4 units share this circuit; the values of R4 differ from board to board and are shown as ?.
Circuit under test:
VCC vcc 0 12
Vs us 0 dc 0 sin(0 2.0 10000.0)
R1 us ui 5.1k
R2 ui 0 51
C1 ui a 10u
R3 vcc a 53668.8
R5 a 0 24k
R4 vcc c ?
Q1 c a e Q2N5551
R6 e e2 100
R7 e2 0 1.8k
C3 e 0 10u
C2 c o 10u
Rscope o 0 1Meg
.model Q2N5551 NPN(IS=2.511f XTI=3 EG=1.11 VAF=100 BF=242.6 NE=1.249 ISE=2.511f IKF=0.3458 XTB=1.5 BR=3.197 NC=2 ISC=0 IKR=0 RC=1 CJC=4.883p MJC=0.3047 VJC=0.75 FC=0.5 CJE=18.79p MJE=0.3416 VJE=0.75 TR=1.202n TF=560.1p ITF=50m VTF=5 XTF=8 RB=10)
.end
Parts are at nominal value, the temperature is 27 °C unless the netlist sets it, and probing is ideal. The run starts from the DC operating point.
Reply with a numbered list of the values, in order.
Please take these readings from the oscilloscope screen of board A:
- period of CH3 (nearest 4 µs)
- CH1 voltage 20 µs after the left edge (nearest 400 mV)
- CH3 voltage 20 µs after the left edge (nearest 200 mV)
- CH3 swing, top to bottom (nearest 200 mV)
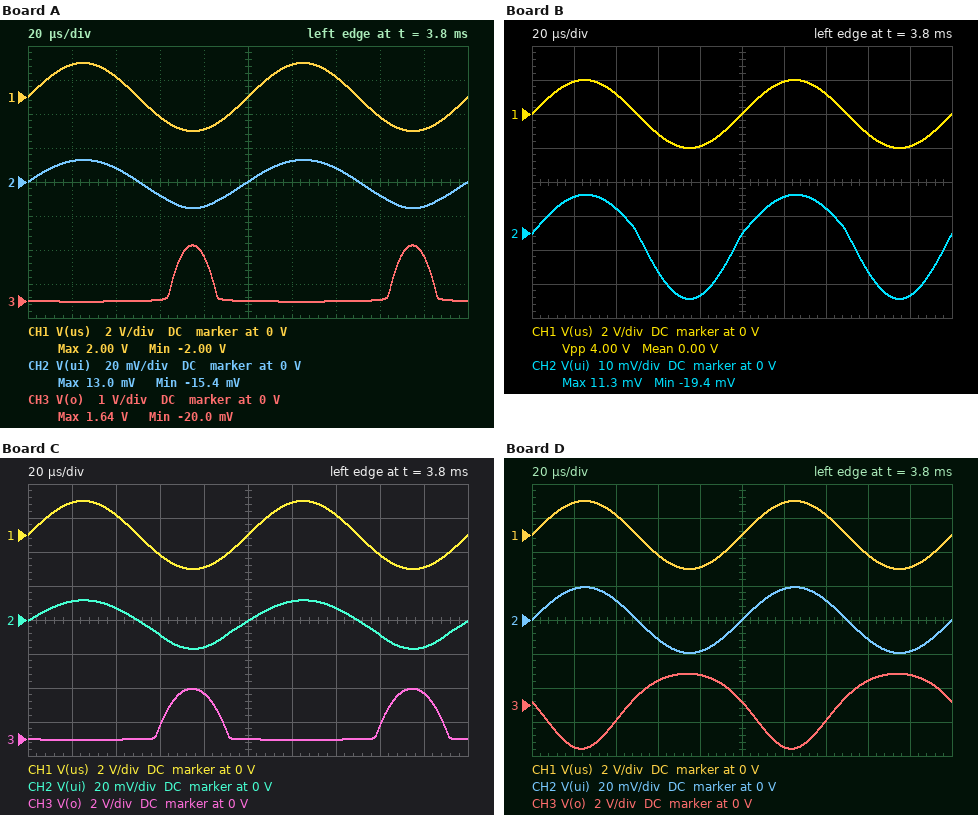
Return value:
1. 100 µs
2. 2.0 V
3. 0 V
4. 1.6 V
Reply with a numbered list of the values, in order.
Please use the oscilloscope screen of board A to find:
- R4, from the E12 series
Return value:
1. 15 kΩ
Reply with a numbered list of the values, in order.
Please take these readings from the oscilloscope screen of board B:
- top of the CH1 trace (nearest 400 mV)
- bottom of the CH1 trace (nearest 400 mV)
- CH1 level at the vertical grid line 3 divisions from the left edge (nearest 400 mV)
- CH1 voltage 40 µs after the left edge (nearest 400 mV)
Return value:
1. 2.0 V
2. -2.0 V
3. -1.2 V
4. 1.2 V
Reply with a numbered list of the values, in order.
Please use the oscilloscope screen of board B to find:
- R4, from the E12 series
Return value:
1. 5.6 kΩ
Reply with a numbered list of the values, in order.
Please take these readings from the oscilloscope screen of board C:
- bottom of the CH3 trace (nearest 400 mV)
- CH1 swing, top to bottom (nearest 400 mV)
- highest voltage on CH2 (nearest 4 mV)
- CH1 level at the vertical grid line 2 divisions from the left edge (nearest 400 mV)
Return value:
1. 0 V
2. 4.0 V
3. 12 mV
4. 1.2 V
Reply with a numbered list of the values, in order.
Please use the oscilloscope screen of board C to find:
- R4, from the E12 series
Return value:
1. 10 kΩ
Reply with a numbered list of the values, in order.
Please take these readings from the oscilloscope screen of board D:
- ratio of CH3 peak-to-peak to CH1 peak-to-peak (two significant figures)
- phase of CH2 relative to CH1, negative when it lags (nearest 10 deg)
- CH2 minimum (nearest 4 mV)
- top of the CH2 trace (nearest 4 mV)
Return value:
1. 1.1
2. 0 deg
3. -20 mV
4. 20 mV
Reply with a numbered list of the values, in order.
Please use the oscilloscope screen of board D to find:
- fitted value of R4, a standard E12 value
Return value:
1. 2.2 kΩ
